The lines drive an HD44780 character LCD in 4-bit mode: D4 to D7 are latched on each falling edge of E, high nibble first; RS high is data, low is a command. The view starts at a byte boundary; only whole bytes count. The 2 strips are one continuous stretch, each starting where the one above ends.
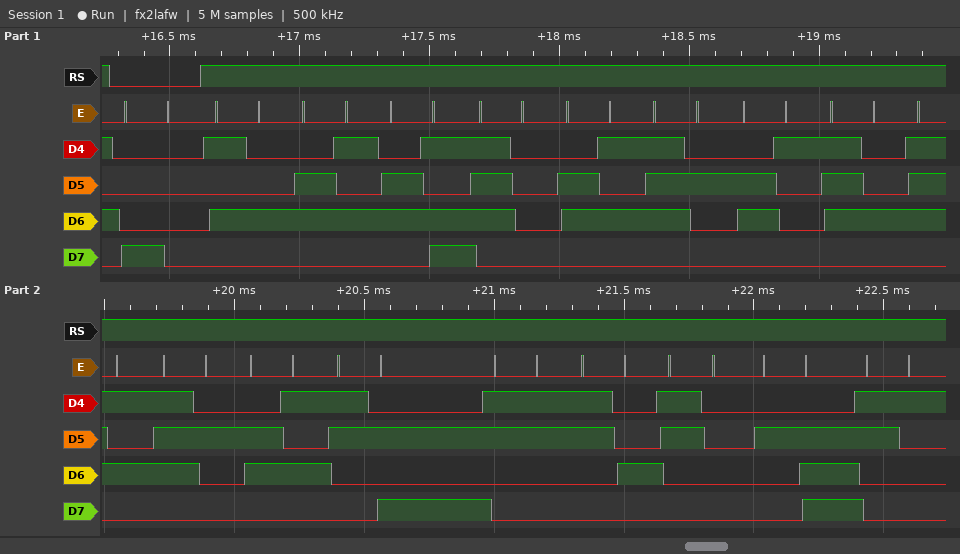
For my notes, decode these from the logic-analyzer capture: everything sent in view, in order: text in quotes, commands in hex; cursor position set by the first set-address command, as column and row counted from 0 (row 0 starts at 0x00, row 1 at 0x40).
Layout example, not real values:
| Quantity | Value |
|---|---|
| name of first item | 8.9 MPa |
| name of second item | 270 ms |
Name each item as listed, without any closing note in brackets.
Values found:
| Quantity | Value |
|---|---|
| everything sent in view, in order: text in quotes, commands in hex | 0x80 "Temperature:340.1" |
| cursor position set by the first set-address command, as column and row counted from 0 | column 0, row 0 |
